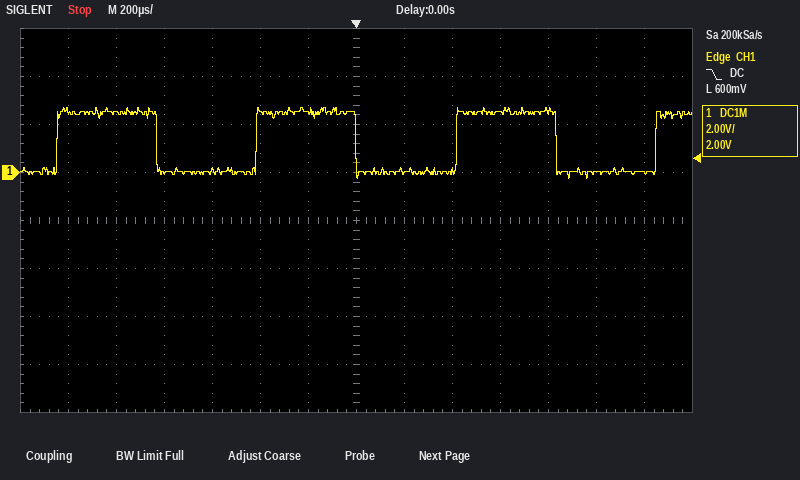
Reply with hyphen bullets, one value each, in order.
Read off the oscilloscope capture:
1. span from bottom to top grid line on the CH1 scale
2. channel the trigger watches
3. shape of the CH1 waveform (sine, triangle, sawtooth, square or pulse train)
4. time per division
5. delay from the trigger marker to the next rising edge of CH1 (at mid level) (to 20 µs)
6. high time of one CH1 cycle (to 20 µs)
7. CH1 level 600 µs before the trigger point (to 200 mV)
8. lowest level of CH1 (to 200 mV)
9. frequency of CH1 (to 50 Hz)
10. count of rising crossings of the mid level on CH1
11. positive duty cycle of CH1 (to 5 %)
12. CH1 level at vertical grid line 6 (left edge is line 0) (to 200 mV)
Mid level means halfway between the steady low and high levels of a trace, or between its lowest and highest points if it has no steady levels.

- 16 V
- CH1
- square
- 200 µs
- 420 µs
- 420 µs
- 0.0 V
- -200 mV
- 1.20 kHz
- 4
- 50 %
- 2.4 V
